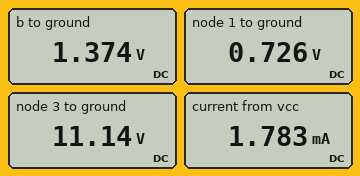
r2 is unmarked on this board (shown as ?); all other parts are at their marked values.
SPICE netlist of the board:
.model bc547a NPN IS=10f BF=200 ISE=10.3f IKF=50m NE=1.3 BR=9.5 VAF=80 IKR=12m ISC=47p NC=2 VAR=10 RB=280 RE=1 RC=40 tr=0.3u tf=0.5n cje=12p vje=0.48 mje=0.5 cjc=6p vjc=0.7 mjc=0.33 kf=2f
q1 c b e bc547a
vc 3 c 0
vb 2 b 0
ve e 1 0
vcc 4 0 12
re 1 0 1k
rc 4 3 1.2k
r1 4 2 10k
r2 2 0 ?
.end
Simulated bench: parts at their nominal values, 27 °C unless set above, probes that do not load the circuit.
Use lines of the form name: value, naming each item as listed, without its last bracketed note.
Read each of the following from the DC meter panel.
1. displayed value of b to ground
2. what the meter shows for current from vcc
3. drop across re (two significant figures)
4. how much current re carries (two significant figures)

displayed value of b to ground: 1.374 V
what the meter shows for current from vcc: 1.783 mA
drop across re: 730 mV
how much current re carries: 730 µA
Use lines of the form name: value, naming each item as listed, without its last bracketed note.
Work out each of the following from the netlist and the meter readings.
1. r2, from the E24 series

r2, from the E24 series: 1.3 kΩ
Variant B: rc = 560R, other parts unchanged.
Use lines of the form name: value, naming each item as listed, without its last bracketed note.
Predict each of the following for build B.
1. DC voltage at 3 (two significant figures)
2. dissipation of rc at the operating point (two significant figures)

DC voltage at 3: 12 V
dissipation of rc at the operating point: 290 µW
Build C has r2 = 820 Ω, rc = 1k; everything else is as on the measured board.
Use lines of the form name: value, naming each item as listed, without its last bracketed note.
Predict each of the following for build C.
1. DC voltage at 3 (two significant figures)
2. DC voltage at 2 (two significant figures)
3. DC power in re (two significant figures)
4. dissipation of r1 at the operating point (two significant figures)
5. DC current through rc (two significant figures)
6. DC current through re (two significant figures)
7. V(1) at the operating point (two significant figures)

DC voltage at 3: 12 V
DC voltage at 2: 910 mV
DC power in re: 82 µW
dissipation of r1 at the operating point: 12 mW
DC current through rc: 280 µA
DC current through re: 290 µA
V(1) at the operating point: 290 mV
